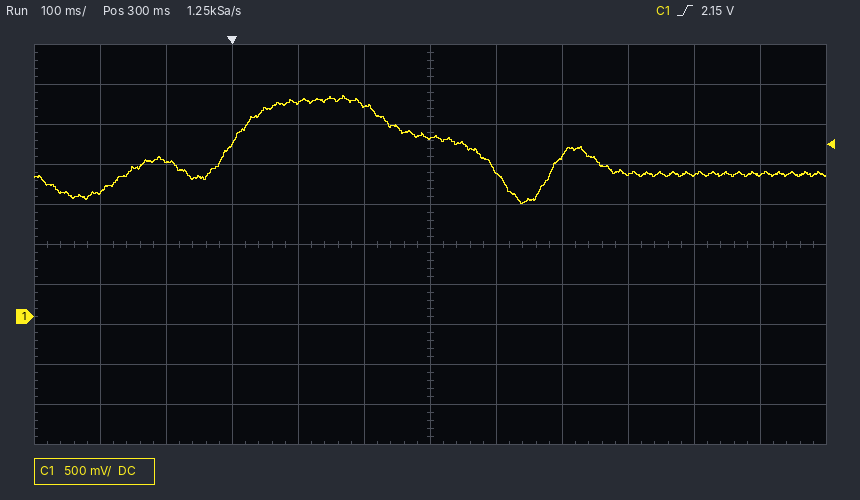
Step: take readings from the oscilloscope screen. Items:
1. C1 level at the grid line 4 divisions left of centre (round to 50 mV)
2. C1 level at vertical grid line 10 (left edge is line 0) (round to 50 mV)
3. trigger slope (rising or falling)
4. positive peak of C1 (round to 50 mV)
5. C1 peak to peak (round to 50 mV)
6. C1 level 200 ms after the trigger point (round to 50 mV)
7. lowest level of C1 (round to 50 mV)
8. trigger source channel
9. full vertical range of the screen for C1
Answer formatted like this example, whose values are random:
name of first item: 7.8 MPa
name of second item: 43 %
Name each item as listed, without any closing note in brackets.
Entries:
C1 level at the grid line 4 divisions left of centre: 1.95 V
C1 level at vertical grid line 10 (left edge is line 0): 1.75 V
trigger slope: rising
positive peak of C1: 2.75 V
C1 peak to peak: 1.35 V
C1 level 200 ms after the trigger point: 2.65 V
lowest level of C1: 1.40 V
trigger source channel: C1
full vertical range of the screen for C1: 5 V
